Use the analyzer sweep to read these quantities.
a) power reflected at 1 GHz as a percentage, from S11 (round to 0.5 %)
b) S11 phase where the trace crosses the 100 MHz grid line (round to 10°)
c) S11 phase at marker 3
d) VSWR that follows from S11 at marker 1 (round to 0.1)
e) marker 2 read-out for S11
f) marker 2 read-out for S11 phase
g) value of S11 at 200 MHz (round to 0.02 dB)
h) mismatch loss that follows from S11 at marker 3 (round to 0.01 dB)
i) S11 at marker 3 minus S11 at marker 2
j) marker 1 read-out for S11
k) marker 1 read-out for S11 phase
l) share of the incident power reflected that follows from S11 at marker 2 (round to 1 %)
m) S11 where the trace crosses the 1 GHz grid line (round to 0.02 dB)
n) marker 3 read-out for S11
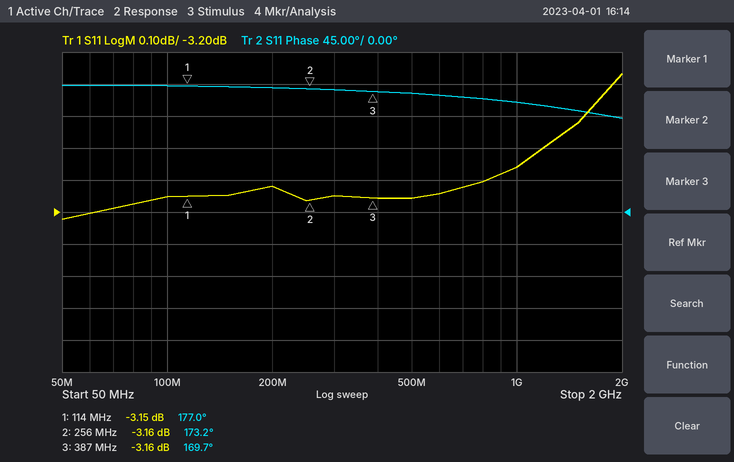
49.5 %
180°
169.7°
5.6
-3.16 dB
173.2°
-3.12 dB
2.87 dB
0.00 dB
-3.15 dB
177.0°
48 %
-3.06 dB
-3.16 dB
